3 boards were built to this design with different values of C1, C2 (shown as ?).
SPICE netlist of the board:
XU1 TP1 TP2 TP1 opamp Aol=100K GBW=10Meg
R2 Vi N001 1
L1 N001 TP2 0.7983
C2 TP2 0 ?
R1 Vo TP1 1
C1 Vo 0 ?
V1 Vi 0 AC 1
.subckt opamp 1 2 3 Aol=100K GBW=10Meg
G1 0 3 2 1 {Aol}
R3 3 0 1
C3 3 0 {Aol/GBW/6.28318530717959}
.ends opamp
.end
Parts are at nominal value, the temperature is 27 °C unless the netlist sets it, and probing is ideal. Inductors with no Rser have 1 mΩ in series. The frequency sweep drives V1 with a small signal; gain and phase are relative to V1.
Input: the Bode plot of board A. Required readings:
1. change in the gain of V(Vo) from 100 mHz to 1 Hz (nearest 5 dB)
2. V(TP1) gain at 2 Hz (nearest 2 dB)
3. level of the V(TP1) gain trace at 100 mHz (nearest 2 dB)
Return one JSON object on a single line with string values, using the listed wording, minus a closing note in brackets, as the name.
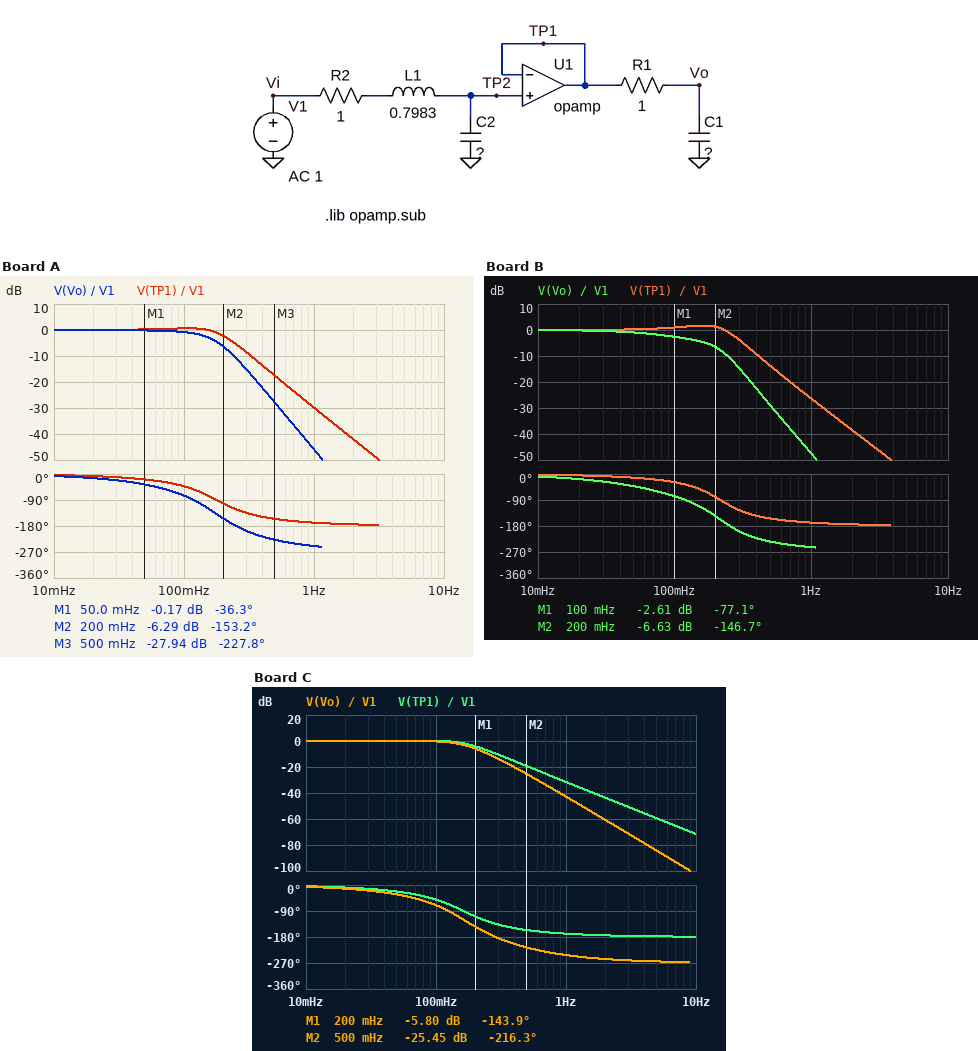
{"change in the gain of V(Vo) from 100 mHz to 1 Hz": "-45 dB", "V(TP1) gain at 2 Hz": "-42 dB", "level of the V(TP1) gain trace at 100 mHz": "0 dB"}
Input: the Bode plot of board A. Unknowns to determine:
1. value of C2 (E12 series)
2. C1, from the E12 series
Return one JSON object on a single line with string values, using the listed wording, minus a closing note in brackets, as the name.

{"value of C2": "1 F", "C1, from the E12 series": "1 F"}
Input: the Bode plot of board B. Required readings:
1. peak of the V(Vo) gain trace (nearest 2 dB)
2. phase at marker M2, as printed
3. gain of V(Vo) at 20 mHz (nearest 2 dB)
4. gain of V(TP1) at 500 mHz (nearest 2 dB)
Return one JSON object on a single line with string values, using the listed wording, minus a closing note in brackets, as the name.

{"peak of the V(Vo) gain trace": "0 dB", "phase at marker M2, as printed": "-146.7 deg", "gain of V(Vo) at 20 mHz": "0 dB", "gain of V(TP1) at 500 mHz": "-14 dB"}
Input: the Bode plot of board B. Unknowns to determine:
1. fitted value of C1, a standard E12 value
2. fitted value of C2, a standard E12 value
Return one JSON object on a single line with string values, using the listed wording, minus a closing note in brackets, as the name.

{"fitted value of C1, a standard E12 value": "1.8 F", "fitted value of C2, a standard E12 value": "680 mF"}
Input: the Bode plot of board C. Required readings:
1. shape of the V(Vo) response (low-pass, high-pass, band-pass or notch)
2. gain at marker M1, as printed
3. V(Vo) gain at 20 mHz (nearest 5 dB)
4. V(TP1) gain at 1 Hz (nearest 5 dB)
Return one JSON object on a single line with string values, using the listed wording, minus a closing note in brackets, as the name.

{"shape of the V(Vo) response": "low-pass", "gain at marker M1, as printed": "-5.80 dB", "V(Vo) gain at 20 mHz": "0 dB", "V(TP1) gain at 1 Hz": "-30 dB"}
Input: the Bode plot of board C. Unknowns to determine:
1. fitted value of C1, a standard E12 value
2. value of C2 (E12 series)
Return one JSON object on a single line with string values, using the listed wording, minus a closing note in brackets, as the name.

{"fitted value of C1, a standard E12 value": "560 mF", "value of C2": "1.2 F"}
